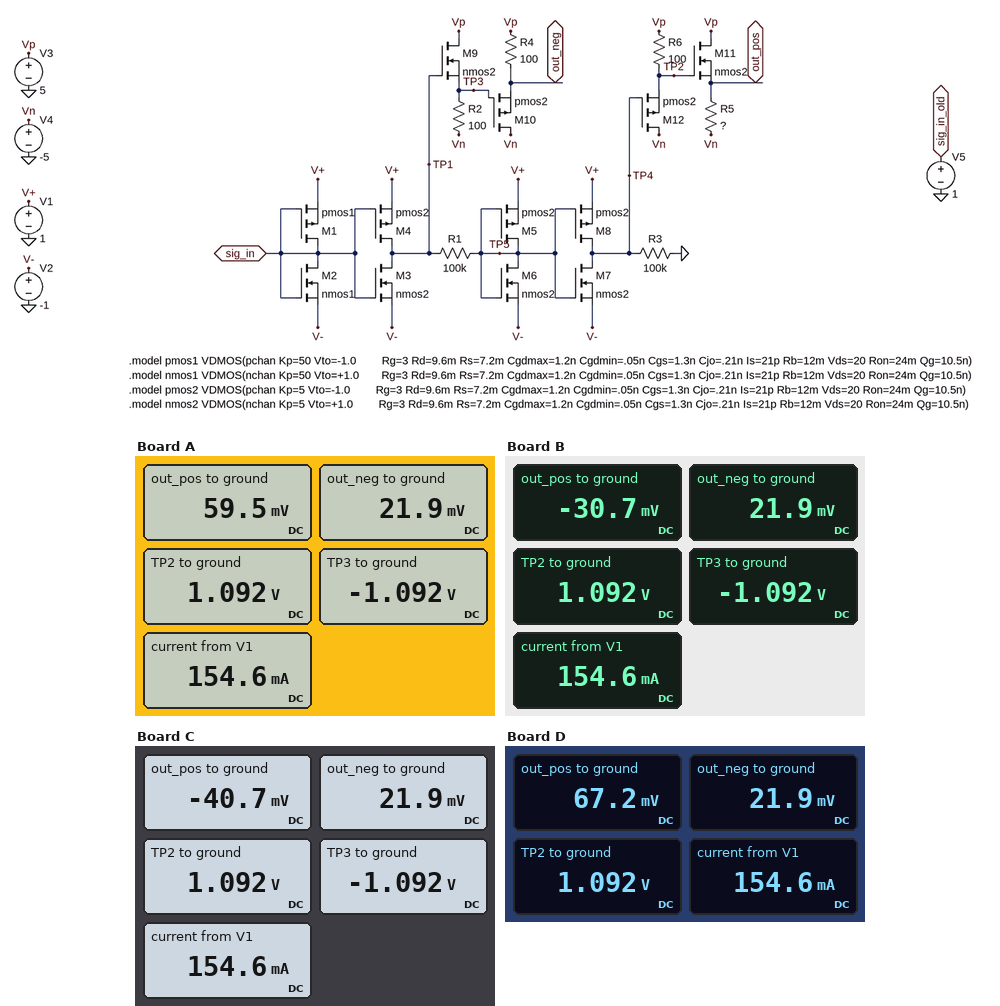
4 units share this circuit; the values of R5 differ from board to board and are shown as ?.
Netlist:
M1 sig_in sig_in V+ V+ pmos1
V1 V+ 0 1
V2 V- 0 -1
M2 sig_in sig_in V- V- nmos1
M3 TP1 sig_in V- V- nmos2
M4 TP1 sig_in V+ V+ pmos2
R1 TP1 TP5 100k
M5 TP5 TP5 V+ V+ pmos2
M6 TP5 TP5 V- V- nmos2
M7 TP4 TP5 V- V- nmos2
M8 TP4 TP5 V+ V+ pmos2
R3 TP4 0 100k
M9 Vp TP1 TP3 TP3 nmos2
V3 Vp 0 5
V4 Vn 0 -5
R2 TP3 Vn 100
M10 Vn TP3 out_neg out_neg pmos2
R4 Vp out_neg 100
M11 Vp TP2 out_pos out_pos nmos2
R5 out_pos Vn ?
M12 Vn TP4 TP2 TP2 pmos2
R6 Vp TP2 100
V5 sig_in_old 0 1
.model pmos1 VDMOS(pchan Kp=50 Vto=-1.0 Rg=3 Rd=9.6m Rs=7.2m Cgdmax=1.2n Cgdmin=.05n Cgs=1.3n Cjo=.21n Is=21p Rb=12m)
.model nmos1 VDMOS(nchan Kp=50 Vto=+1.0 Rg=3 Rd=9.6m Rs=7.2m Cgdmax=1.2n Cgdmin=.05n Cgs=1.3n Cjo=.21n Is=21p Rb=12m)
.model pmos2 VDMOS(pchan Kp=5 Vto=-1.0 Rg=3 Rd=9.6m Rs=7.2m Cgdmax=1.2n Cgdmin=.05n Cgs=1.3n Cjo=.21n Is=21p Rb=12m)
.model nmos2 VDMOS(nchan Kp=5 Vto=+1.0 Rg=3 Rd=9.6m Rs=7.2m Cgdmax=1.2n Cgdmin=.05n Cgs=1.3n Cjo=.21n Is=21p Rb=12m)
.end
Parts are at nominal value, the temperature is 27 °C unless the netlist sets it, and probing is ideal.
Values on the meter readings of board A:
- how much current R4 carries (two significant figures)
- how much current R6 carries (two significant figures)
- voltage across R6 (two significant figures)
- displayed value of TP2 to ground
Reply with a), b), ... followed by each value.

a) 50 mA
b) 39 mA
c) 3.9 V
d) 1.092 V
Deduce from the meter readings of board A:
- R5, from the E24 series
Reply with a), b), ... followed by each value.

a) 270 Ω
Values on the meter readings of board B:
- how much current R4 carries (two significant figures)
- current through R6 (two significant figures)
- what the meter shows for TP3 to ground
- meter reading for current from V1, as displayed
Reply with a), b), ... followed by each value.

a) 50 mA
b) 39 mA
c) -1.092 V
d) 154.6 mA
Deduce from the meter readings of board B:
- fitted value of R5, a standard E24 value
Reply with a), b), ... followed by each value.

a) 91 Ω
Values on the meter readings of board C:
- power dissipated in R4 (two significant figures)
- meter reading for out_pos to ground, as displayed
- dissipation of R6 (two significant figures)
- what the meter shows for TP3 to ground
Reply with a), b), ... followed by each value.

a) 250 mW
b) -40.7 mV
c) 150 mW
d) -1.092 V
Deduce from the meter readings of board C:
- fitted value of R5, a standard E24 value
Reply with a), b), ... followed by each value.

a) 82 Ω
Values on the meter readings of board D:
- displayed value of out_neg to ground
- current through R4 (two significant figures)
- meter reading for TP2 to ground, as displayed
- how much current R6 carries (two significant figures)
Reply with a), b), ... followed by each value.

a) 21.9 mV
b) 50 mA
c) 1.092 V
d) 39 mA
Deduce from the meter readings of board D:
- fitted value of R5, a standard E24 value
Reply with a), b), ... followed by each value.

a) 300 Ω
